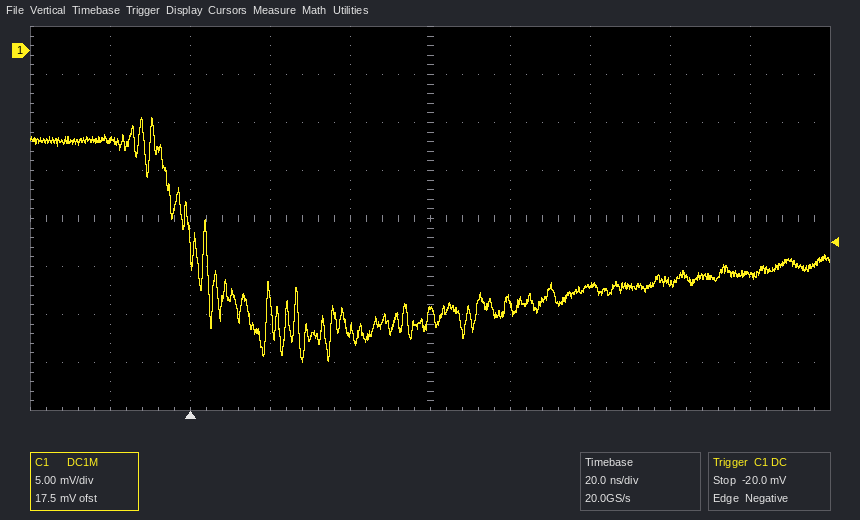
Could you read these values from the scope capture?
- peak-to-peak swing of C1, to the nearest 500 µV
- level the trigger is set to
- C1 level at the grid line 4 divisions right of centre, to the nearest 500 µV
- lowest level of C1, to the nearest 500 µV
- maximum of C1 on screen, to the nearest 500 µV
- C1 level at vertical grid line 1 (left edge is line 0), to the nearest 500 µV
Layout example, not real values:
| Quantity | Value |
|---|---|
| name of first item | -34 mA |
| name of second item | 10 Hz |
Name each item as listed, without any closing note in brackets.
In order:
| Quantity | Value |
|---|---|
| peak-to-peak swing of C1, to the nearest 500 µV | 25.5 mV |
| level the trigger is set to | -20.0 mV |
| C1 level at the grid line 4 divisions right of centre, to the nearest 500 µV | -23.5 mV |
| lowest level of C1, to the nearest 500 µV | -32.5 mV |
| maximum of C1 on screen, to the nearest 500 µV | -7.0 mV |
| C1 level at vertical grid line 1 (left edge is line 0), to the nearest 500 µV | -9.5 mV |
